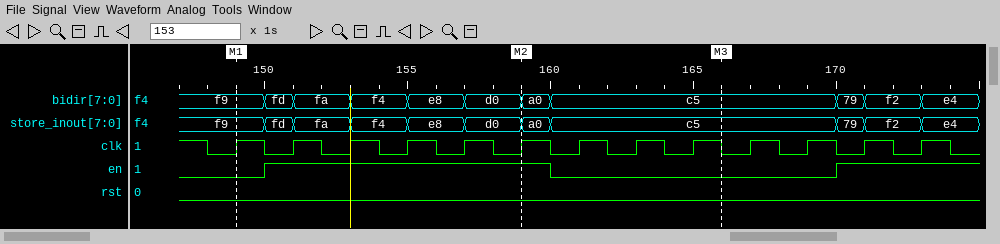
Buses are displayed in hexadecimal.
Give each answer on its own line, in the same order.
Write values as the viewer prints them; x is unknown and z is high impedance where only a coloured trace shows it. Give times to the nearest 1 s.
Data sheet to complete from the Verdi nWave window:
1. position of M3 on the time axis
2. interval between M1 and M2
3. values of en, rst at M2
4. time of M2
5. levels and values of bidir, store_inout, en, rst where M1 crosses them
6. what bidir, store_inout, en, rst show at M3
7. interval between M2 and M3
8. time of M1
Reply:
166 s
10 s
en=1, rst=0
159 s
bidir=f9, store_inout=f9, en=0, rst=0
bidir=c5, store_inout=c5, en=0, rst=0
7 s
149 s
